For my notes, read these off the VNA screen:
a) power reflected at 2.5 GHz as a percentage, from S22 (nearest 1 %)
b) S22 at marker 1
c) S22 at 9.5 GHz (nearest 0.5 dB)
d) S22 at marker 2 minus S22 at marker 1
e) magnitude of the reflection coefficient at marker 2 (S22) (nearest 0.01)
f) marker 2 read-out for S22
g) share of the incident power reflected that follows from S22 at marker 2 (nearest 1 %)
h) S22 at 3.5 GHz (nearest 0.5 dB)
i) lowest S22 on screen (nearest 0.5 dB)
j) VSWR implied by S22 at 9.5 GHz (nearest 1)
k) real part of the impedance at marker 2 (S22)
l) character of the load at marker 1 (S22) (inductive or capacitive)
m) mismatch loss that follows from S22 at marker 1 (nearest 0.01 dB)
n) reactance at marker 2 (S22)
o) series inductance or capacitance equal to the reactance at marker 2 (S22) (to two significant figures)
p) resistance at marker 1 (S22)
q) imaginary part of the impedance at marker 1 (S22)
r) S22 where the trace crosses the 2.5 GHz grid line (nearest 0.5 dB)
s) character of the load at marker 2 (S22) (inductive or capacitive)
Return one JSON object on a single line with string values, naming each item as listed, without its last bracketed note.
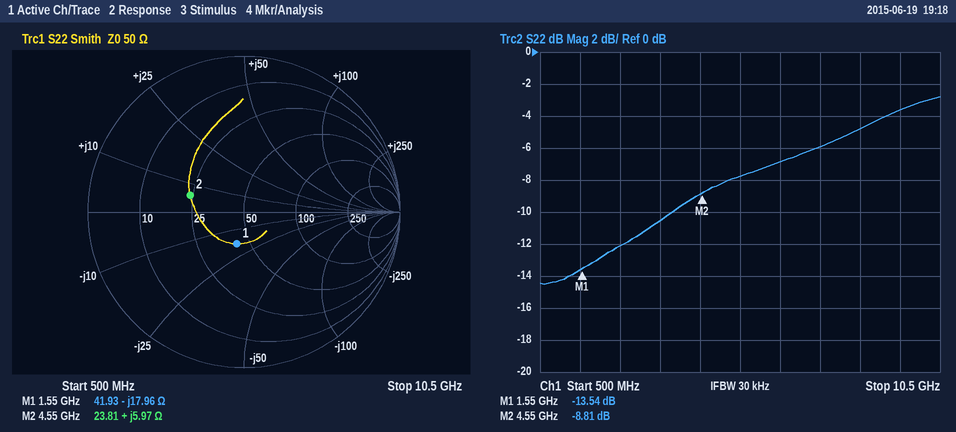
{"power reflected at 2.5 GHz as a percentage, from S22": "6 %", "S22 at marker 1": "-13.54 dB", "S22 at 9.5 GHz": "-3.5 dB", "S22 at marker 2 minus S22 at marker 1": "4.73 dB", "magnitude of the reflection coefficient at marker 2 (S22)": "0.36", "marker 2 read-out for S22": "-8.81 dB", "share of the incident power reflected that follows from S22 at marker 2": "13 %", "S22 at 3.5 GHz": "-10.5 dB", "lowest S22 on screen": "-14.5 dB", "VSWR implied by S22 at 9.5 GHz": "5", "real part of the impedance at marker 2": "23.81 Ω", "character of the load at marker 1 (S22)": "capacitive", "mismatch loss that follows from S22 at marker 1": "0.20 dB", "reactance at marker 2": "+5.97 Ω", "series inductance or capacitance equal to the reactance at marker 2 (S22)": "210 pH", "resistance at marker 1": "41.93 Ω", "imaginary part of the impedance at marker 1": "-17.96 Ω", "S22 where the trace crosses the 2.5 GHz grid line": "-12.0 dB", "character of the load at marker 2 (S22)": "inductive"}
